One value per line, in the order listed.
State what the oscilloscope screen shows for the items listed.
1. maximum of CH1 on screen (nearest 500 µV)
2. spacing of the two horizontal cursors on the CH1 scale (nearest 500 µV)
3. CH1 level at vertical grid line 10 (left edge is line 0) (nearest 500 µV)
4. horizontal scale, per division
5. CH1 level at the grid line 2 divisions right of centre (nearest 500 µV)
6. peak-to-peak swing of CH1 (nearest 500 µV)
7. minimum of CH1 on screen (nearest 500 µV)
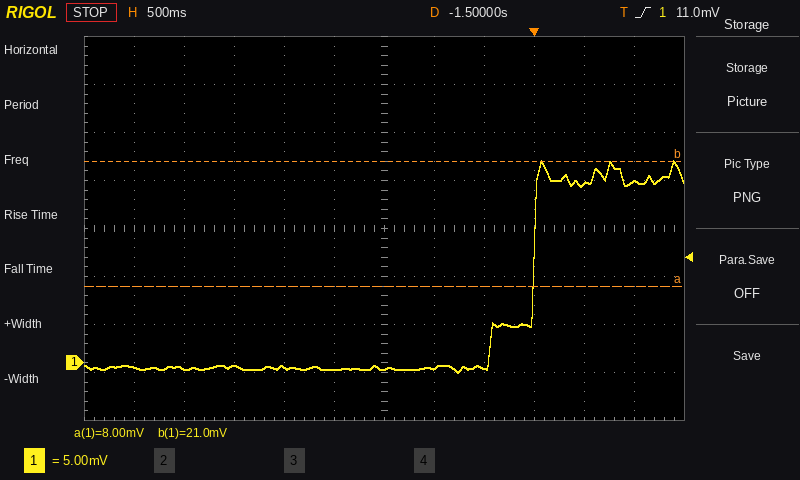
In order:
21.0 mV
13.0 mV
18.5 mV
500 ms
-500 µV
22.0 mV
-1.0 mV
